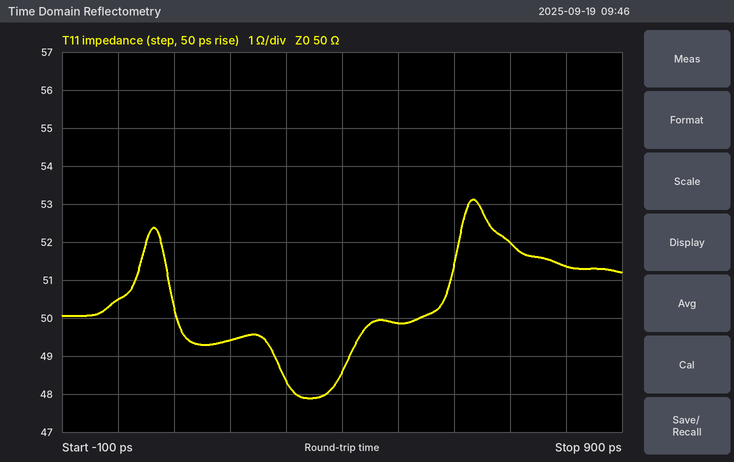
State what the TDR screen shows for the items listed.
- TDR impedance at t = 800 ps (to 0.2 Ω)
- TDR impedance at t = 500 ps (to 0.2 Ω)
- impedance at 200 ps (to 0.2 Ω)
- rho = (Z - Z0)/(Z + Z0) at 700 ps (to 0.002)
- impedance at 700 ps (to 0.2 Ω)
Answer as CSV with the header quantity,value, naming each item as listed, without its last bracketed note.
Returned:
quantity,value
TDR impedance at t = 800 ps,51.4 Ω
TDR impedance at t = 500 ps,49.8 Ω
impedance at 200 ps,49.4 Ω
rho = (Z - Z0)/(Z + Z0) at 700 ps,+0.020
impedance at 700 ps,52.0 Ω
